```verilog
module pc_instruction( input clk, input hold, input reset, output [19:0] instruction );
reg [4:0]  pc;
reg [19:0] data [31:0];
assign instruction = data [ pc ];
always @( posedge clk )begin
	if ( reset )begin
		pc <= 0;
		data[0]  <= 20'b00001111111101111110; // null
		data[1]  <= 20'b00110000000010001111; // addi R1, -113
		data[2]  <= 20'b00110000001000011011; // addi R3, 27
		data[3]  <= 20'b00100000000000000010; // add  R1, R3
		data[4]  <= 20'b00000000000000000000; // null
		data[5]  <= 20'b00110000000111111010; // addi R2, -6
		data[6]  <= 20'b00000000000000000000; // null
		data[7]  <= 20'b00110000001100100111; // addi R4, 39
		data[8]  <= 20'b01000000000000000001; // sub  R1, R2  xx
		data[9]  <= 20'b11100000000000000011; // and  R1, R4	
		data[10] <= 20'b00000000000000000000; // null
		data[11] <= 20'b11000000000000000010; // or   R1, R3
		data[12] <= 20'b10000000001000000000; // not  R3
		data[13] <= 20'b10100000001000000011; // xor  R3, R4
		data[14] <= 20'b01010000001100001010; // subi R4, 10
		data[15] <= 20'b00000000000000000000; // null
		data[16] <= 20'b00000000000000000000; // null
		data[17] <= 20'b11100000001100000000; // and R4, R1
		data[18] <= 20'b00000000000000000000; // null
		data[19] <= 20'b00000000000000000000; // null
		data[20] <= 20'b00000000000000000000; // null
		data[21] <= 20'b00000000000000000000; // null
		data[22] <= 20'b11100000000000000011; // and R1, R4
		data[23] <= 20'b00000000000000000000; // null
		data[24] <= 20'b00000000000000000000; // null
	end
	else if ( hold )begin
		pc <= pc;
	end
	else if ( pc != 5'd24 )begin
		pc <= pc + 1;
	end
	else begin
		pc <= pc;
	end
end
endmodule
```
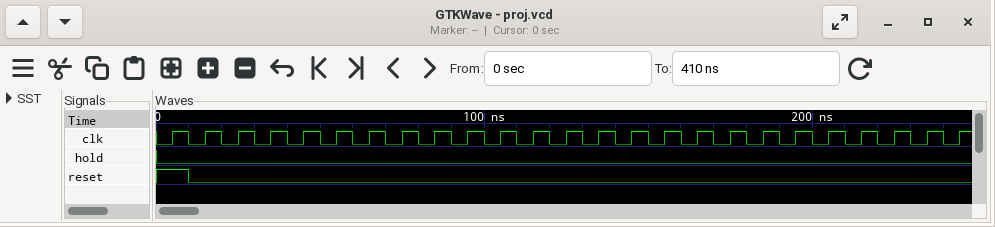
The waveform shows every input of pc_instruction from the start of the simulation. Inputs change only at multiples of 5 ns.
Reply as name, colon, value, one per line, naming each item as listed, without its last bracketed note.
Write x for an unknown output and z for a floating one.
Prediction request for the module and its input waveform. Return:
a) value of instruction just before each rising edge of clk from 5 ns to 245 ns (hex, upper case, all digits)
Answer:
value of instruction just before each rising edge of clk from 5 ns to 245 ns: x, 0FF7E, 3008F, 3021B, 20002, 00000, 301FA, 00000, 30327, 40001, E0003, 00000, C0002, 80200, A0203, 5030A, 00000, 00000, E0300, 00000, 00000, 00000, 00000, E0003, 00000
